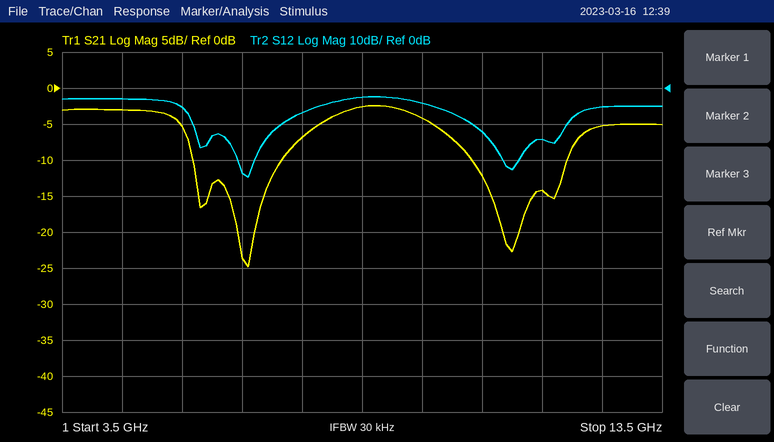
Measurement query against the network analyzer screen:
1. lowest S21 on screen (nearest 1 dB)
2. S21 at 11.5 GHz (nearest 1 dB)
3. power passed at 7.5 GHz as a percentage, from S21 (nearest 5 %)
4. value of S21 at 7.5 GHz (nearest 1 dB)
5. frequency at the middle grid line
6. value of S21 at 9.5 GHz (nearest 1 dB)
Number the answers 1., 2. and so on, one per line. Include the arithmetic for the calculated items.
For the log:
1. -25 dB
2. -14 dB
3. 10^(-7/10) ≈ 20 %
4. -7 dB
5. 8.5 GHz
6. -4 dB
